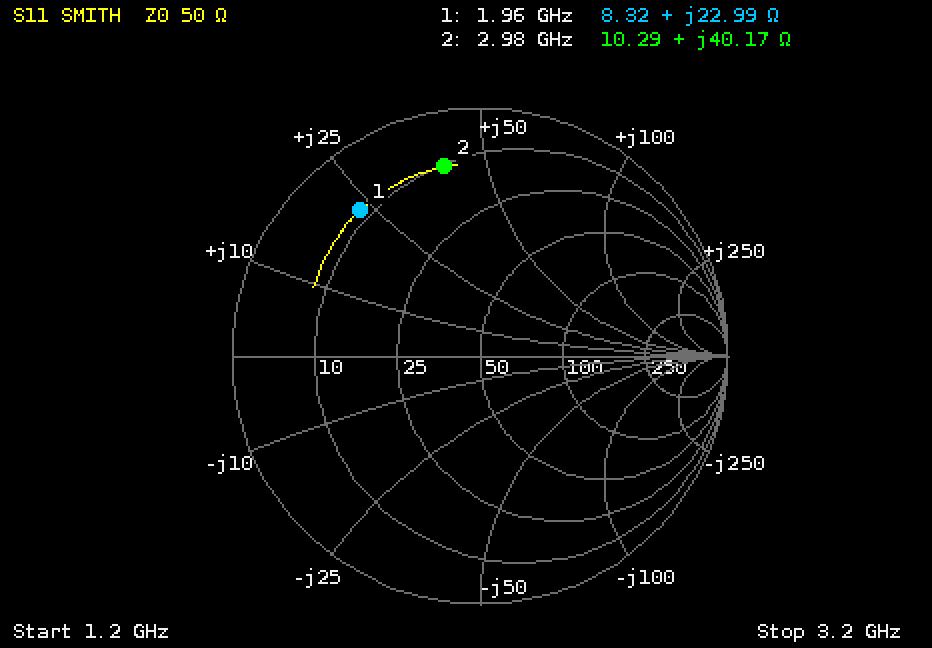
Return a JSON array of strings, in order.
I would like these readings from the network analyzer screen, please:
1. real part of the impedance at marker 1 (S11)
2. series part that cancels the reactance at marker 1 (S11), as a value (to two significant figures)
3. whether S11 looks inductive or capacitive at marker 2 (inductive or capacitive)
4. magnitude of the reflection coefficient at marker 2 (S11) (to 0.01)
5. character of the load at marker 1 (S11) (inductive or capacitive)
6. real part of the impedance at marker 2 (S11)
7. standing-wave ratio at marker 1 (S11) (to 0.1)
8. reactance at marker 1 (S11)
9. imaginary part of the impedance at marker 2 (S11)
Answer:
["8.32 Ω", "3.5 pF", "inductive", "0.78", "inductive", "10.29 Ω", "7.3", "+22.99 Ω", "+40.17 Ω"]
